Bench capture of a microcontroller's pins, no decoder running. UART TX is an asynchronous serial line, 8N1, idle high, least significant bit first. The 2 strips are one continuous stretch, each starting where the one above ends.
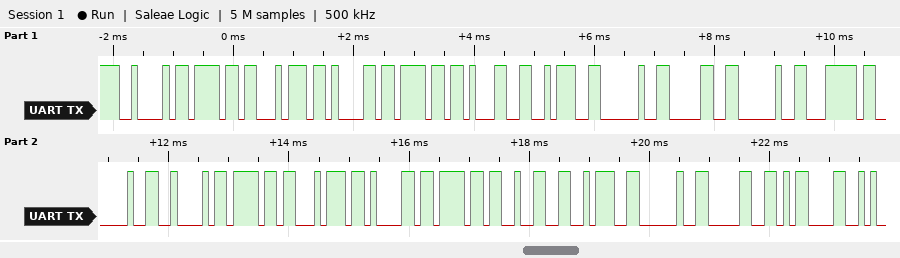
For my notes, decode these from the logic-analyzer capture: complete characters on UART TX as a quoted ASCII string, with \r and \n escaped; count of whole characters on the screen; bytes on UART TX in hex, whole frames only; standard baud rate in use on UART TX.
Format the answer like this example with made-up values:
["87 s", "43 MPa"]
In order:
["\"Botao1: 0 | Botao2: 0\\r\"", "22", "42 6F 74 61 6F 31 3A 20 30 20 7C 20 42 6F 74 61 6F 32 3A 20 30 0D", "9600 baud"]
